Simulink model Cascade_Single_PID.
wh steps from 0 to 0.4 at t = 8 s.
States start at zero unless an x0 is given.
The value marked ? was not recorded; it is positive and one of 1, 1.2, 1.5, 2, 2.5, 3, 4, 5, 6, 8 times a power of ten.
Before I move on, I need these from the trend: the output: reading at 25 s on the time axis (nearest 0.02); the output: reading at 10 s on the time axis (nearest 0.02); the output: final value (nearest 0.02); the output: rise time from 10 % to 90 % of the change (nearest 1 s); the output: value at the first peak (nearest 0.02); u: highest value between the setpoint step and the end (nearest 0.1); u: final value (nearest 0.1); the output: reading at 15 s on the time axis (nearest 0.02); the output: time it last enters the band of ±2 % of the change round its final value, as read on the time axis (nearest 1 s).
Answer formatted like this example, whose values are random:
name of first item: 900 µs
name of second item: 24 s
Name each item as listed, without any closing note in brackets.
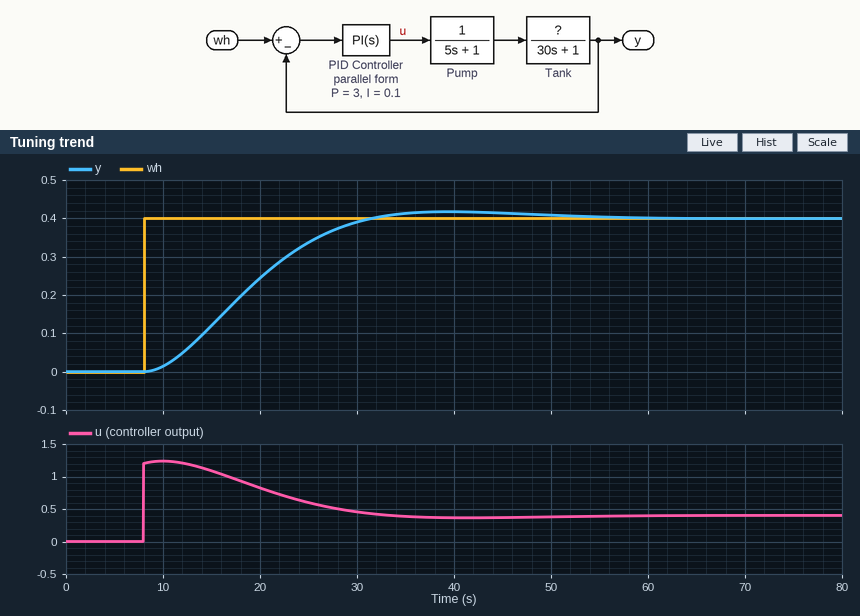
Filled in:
the output: reading at 25 s on the time axis: 0.34
the output: reading at 10 s on the time axis: 0.02
the output: final value: 0.40
the output: rise time from 10 % to 90 % of the change: 15 s
the output: value at the first peak: 0.42
u: highest value between the setpoint step and the end: 1.2
u: final value: 0.4
the output: reading at 15 s on the time axis: 0.12
the output: time it last enters the band of ±2 % of the change round its final value, as read on the time axis: 50 s
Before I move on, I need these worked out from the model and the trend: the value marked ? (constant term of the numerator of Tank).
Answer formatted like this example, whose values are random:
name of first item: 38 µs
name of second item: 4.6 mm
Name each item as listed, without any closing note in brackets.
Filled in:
the value marked ?: 1
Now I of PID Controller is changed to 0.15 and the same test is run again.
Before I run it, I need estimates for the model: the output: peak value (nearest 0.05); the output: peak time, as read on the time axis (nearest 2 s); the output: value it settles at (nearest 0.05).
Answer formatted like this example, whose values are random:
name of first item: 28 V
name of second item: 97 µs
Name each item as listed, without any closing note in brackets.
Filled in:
the output: peak value: 0.45
the output: peak time, as read on the time axis: 38 s
the output: value it settles at: 0.40
